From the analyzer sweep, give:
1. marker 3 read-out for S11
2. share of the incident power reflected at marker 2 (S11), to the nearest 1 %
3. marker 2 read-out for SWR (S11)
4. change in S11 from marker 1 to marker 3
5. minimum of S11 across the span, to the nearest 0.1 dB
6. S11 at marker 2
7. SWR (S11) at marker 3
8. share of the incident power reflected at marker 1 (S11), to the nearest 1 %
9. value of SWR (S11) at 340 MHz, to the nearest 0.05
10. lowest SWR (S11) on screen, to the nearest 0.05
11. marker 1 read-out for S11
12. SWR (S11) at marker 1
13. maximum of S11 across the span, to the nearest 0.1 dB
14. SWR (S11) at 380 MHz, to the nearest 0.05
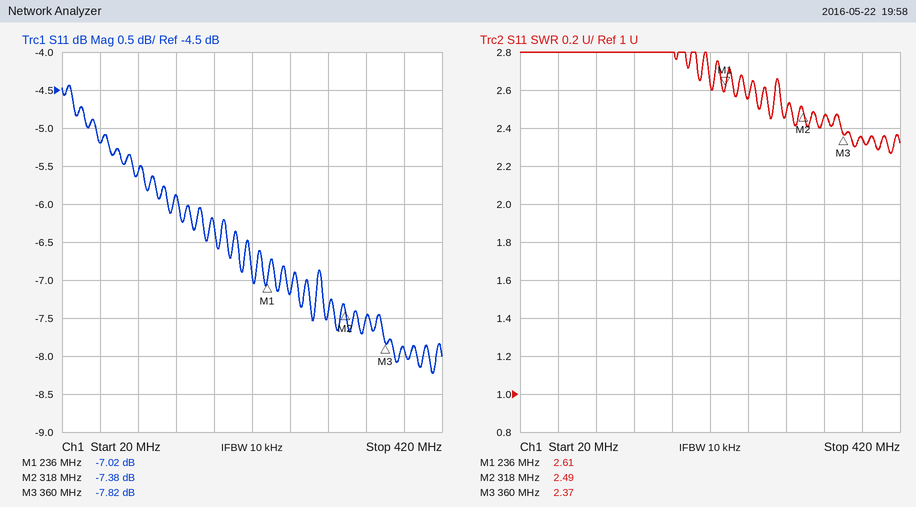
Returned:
-7.82 dB
18 %
2.49
-0.80 dB
-8.2 dB
-7.38 dB
2.37
20 %
2.45
2.25
-7.02 dB
2.61
-4.4 dB
2.35
